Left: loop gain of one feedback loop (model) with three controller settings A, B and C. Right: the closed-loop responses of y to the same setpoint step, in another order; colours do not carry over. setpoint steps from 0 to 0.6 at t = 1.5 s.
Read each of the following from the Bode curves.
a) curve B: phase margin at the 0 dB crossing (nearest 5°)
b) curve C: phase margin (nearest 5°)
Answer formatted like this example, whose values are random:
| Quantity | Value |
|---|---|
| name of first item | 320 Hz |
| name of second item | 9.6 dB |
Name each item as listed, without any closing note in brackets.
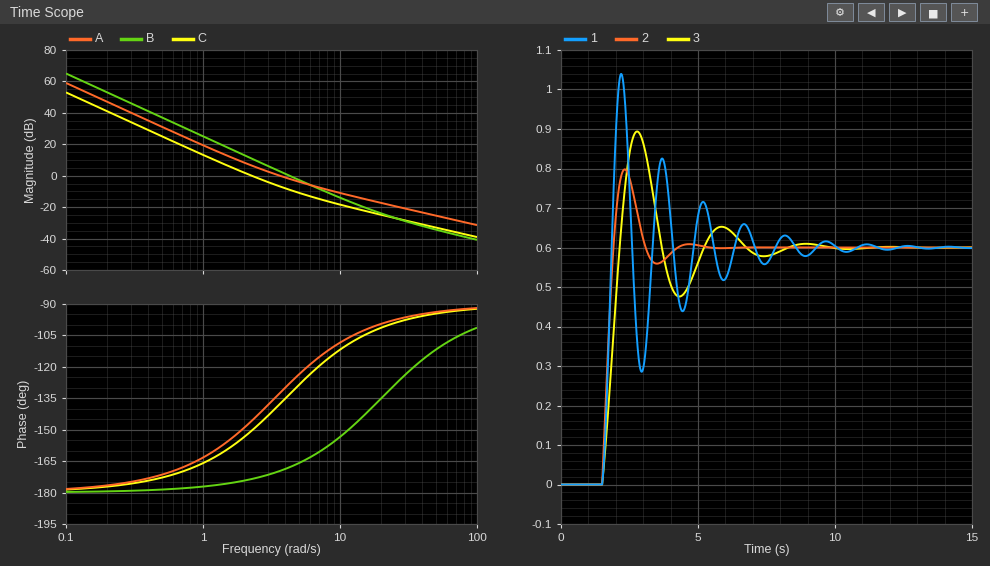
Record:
| Quantity | Value |
|---|---|
| curve B: phase margin at the 0 dB crossing | 10° |
| curve C: phase margin | 30° |
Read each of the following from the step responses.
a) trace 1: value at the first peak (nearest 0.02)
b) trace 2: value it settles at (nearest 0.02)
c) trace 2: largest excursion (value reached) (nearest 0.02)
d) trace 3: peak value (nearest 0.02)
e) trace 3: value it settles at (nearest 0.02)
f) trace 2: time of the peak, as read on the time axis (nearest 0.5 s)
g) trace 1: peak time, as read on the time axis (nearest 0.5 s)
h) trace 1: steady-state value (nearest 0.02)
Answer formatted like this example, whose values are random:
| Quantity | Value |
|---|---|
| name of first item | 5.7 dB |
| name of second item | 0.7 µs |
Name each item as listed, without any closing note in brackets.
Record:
| Quantity | Value |
|---|---|
| trace 1: value at the first peak | 1.04 |
| trace 2: value it settles at | 0.60 |
| trace 2: largest excursion (value reached) | 0.80 |
| trace 3: peak value | 0.90 |
| trace 3: value it settles at | 0.60 |
| trace 2: time of the peak, as read on the time axis | 2.5 s |
| trace 1: peak time, as read on the time axis | 2.0 s |
| trace 1: steady-state value | 0.60 |
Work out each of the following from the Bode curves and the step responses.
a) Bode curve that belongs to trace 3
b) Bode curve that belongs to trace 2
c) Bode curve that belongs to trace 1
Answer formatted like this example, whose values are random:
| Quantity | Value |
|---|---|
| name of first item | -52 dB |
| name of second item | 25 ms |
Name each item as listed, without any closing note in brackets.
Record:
| Quantity | Value |
|---|---|
| Bode curve that belongs to trace 3 | C |
| Bode curve that belongs to trace 2 | A |
| Bode curve that belongs to trace 1 | B |
